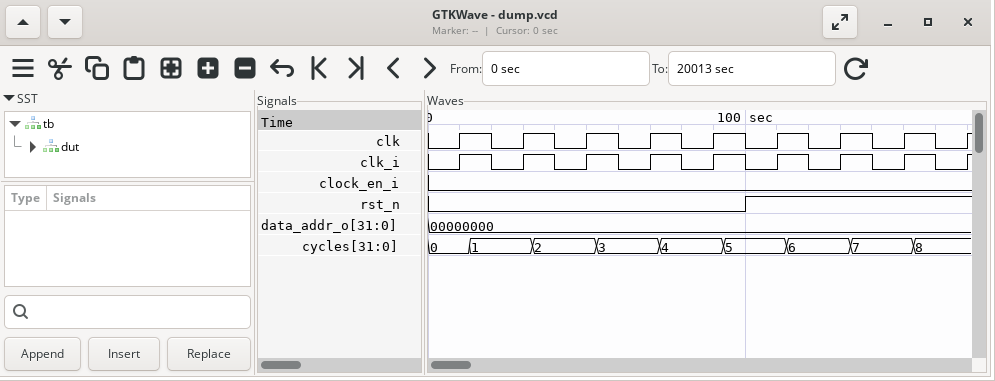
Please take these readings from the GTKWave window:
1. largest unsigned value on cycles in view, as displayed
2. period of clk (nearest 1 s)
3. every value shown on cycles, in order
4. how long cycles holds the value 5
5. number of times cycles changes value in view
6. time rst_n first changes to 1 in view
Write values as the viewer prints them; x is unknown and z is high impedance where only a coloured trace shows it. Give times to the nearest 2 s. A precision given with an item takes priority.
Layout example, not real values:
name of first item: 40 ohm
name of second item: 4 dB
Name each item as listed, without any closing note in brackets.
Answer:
largest unsigned value on cycles in view, as displayed: 8
period of clk: 20 s
every value shown on cycles, in order: 0, 1, 2, 3, 4, 5, 6, 7, 8
how long cycles holds the value 5: 20 s
number of times cycles changes value in view: 8
time rst_n first changes to 1 in view: 100 s
